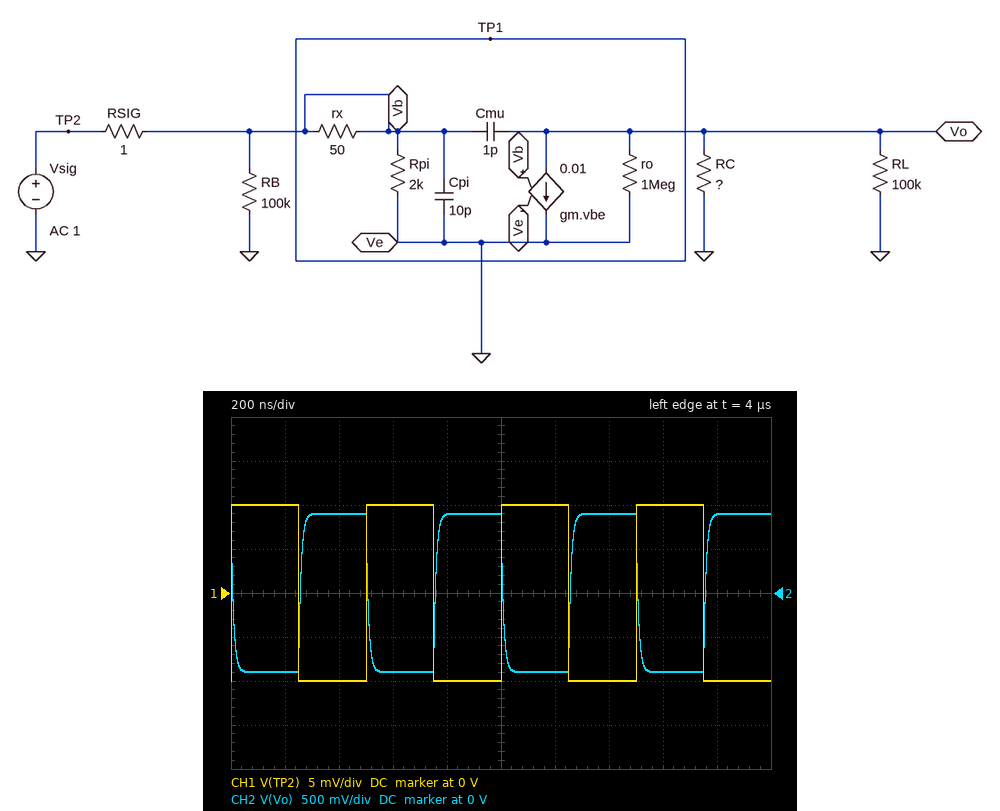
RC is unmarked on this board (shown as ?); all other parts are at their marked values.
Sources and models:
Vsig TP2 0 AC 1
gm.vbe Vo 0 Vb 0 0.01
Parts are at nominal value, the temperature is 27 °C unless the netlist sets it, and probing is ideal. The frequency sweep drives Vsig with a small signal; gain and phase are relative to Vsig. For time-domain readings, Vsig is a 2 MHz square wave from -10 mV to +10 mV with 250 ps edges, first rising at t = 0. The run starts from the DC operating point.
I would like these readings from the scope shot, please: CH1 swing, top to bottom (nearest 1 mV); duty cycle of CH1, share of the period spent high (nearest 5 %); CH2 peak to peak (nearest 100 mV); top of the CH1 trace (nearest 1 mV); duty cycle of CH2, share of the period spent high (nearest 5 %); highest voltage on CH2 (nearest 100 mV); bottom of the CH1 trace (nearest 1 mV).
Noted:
20 mV
50 %
1.8 V
10 mV
50 %
900 mV
-10 mV
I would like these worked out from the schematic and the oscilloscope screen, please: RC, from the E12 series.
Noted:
10 kΩ
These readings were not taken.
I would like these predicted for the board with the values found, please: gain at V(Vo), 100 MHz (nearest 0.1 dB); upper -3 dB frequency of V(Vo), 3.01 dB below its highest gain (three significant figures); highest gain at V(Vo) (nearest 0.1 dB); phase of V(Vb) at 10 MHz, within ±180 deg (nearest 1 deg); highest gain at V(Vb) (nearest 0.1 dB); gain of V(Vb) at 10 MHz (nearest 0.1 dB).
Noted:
23.8 dB
17.5 MHz
39.1 dB
0 deg
0 dB
0 dB
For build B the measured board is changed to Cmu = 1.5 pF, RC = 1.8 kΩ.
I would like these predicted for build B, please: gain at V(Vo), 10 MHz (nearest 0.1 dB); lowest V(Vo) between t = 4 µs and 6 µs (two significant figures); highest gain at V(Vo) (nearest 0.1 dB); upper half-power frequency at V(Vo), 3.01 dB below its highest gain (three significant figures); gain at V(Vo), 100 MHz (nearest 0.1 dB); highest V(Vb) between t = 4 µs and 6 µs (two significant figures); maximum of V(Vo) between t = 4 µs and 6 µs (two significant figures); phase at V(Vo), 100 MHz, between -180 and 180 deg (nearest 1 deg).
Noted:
24.8 dB
-180 mV
24.9 dB
59.7 MHz
19.1 dB
10 mV
180 mV
115 deg
